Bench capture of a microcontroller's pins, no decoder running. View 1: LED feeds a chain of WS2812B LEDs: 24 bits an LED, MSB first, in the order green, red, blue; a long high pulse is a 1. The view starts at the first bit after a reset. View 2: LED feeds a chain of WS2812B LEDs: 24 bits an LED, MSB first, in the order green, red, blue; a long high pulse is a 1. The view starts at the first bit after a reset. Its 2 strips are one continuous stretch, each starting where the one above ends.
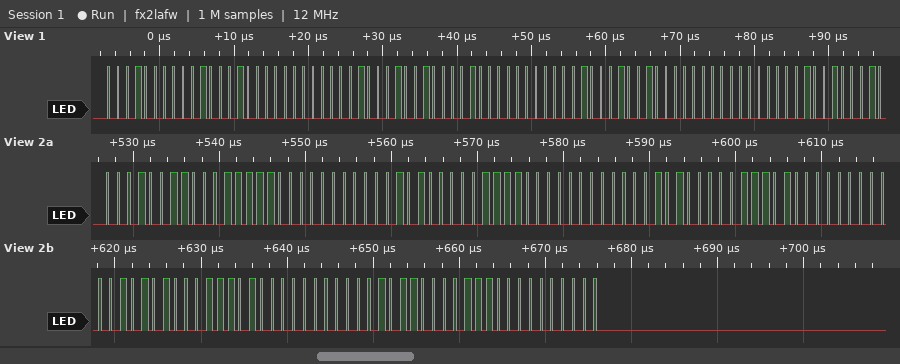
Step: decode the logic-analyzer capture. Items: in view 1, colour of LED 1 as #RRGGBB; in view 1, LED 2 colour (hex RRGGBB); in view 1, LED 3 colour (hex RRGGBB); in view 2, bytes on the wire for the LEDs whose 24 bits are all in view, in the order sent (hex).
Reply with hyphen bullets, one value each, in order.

- #221000
- #211100
- #201100
- 13 1F 00 14 1E 00 14 1D 00 15 1D 00 16 1C 00
